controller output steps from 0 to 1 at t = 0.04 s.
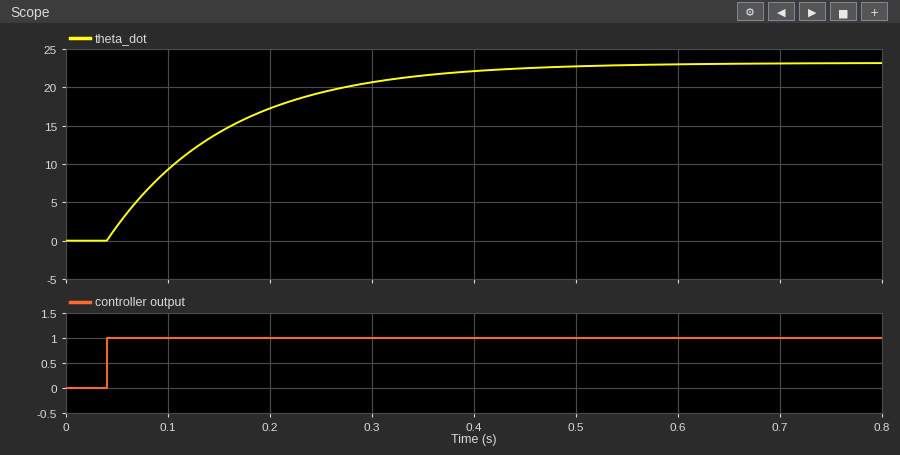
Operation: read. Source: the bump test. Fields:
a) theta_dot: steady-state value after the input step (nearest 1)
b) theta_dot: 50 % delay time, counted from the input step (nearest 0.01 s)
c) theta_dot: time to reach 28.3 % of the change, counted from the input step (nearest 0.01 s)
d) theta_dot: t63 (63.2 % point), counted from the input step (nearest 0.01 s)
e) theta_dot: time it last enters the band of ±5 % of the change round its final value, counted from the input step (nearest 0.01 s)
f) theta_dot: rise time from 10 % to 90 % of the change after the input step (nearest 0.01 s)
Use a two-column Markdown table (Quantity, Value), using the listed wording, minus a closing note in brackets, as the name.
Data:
| Quantity | Value |
|---|---|
| theta_dot: steady-state value after the input step | 23 |
| theta_dot: 50 % delay time, counted from the input step | 0.08 s |
| theta_dot: time to reach 28.3 % of the change, counted from the input step | 0.04 s |
| theta_dot: t63 (63.2 % point), counted from the input step | 0.12 s |
| theta_dot: time it last enters the band of ±5 % of the change round its final value, counted from the input step | 0.35 s |
| theta_dot: rise time from 10 % to 90 % of the change after the input step | 0.26 s |
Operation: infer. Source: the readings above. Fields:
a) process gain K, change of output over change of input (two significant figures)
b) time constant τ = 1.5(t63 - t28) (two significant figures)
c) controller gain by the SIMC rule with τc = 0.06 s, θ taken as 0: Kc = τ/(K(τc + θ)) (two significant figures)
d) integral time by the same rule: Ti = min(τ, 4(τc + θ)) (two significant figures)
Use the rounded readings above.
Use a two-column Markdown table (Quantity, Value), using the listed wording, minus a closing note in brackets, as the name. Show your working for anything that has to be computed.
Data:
| Quantity | Value |
|---|---|
| process gain K, change of output over change of input | (23 - 0) / 1 = 23 |
| time constant τ = 1.5(t63 - t28) | 1.5 × (0.12 - 0.04) = 0.12 s |
| controller gain by the SIMC rule with τc = 0.06 s, θ taken as 0: Kc = τ/(K(τc + θ)) | 0.12 / (23 × (0.06 + 0)) = 0.087 |
| integral time by the same rule: Ti = min(τ, 4(τc + θ)) | min(0.12, 4 × (0.06 + 0)) = 0.12 s |
